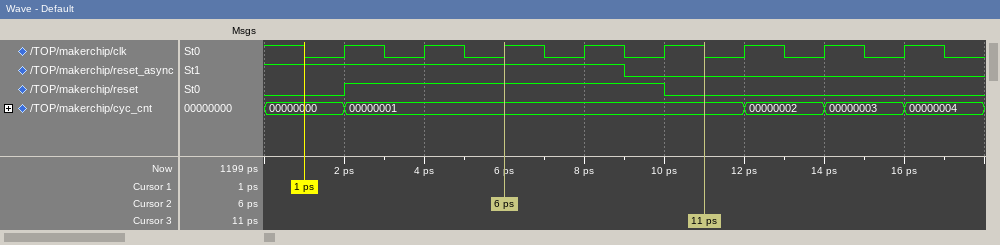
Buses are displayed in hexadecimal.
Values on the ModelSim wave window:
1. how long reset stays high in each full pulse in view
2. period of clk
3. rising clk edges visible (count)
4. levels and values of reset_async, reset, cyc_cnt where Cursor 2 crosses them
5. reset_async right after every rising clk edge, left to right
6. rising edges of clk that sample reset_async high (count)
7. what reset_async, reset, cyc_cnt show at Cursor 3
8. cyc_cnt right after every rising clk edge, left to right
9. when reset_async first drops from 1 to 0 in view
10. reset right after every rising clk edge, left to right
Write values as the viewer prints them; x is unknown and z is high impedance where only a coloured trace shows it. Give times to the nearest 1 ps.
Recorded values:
8 ps
2 ps
8
reset_async=1, reset=1, cyc_cnt=00000001
1 1 1 1 0 0 0 0
4
reset_async=0, reset=0, cyc_cnt=00000001
00000001, 00000001, 00000001, 00000001, 00000001, 00000002, 00000003, 00000004
9 ps
1 1 1 1 0 0 0 0
